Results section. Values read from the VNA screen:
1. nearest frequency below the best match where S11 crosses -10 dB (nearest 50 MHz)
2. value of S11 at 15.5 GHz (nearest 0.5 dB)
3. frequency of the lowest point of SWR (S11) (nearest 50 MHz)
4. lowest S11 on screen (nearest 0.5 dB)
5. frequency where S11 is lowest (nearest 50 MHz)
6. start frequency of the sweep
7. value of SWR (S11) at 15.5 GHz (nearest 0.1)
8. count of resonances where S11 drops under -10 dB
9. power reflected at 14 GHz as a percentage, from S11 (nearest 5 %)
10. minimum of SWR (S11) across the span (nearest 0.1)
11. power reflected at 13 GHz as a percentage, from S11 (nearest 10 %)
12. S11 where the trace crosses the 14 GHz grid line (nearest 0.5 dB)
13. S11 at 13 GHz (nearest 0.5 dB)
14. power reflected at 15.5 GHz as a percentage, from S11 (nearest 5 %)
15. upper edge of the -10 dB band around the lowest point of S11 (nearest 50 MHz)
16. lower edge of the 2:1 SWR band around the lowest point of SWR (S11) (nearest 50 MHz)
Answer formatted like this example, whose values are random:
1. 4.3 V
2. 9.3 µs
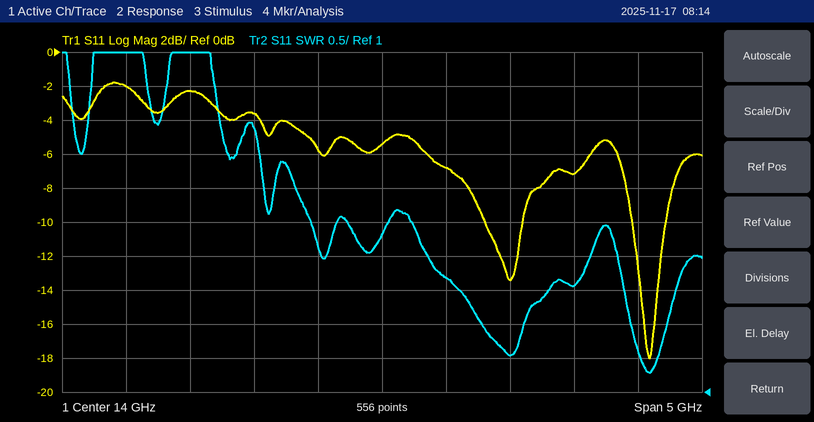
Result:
1. 15.95 GHz
2. -7.0 dB
3. 16.10 GHz
4. -18.0 dB
5. 16.10 GHz
6. 11.5 GHz
7. 2.6
8. 2
9. 30 %
10. 1.3
11. 40 %
12. -5.5 dB
13. -3.5 dB
14. 20 %
15. 16.20 GHz
16. 15.95 GHz
